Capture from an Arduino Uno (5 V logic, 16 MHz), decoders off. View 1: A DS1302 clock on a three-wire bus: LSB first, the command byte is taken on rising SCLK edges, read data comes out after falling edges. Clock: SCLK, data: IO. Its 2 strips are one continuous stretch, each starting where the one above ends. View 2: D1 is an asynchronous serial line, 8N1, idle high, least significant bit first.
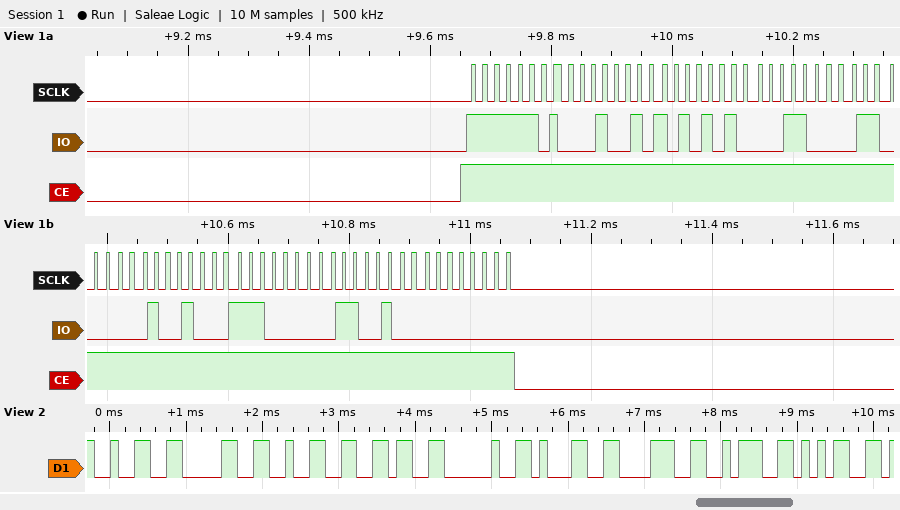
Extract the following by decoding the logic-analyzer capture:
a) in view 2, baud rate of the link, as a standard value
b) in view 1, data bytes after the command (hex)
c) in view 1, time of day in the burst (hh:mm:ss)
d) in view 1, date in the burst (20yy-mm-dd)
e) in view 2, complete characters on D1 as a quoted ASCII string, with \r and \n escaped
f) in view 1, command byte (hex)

9600 baud
48 55 18 06 12 07 26 00
18:55:48
2026-12-06
"2026 18:5"
0xBF
